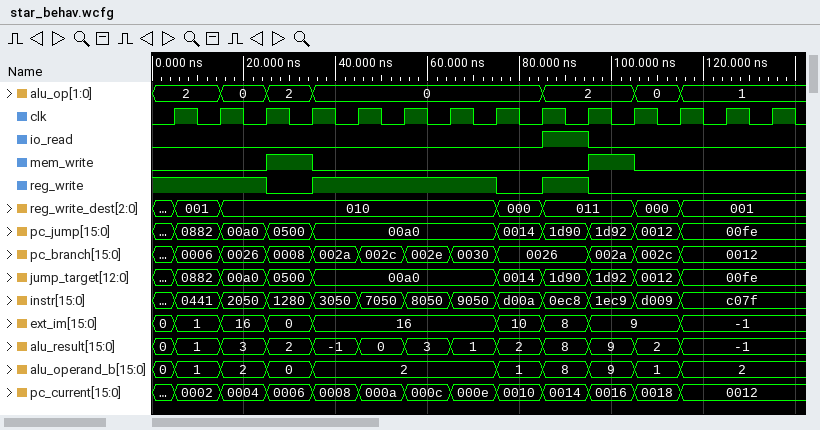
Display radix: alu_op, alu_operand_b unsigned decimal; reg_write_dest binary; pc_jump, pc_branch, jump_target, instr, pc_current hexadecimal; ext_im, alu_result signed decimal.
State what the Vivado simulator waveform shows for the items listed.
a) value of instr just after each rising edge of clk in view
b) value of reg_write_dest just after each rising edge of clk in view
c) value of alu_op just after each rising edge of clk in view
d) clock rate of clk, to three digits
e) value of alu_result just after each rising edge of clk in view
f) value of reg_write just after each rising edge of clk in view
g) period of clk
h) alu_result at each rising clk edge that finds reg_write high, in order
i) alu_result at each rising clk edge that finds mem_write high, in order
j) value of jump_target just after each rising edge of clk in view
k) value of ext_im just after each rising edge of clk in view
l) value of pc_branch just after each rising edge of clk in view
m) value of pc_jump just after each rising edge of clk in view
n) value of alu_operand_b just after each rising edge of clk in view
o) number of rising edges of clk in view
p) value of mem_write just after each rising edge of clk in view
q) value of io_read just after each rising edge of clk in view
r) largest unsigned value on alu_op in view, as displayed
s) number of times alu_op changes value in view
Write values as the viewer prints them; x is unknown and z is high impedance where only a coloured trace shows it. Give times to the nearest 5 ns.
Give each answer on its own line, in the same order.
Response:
0441, 2050, 1280, 3050, 7050, 8050, 9050, d00a, 0ec8, 1ec9, d009, c07f, c07f, c07f
001, 010, 010, 010, 010, 010, 010, 000, 011, 011, 000, 001, 001, 001
2, 0, 2, 0, 0, 0, 0, 0, 2, 2, 0, 1, 1, 1
100 MHz
1, 3, 2, -1, 0, 3, 1, 2, 8, 9, 2, -1, -1, -1
1 1 0 1 1 1 1 0 1 0 0 0 0 0
10 ns
0, 1, 3, -1, 0, 3, 1, 8
2, 9
0882, 00a0, 0500, 00a0, 00a0, 00a0, 00a0, 0014, 1d90, 1d92, 0012, 00fe, 00fe, 00fe
1, 16, 0, 16, 16, 16, 16, 10, 8, 9, 9, -1, -1, -1
0006, 0026, 0008, 002a, 002c, 002e, 0030, 0026, 0026, 002a, 002c, 0012, 0012, 0012
0882, 00a0, 0500, 00a0, 00a0, 00a0, 00a0, 0014, 1d90, 1d92, 0012, 00fe, 00fe, 00fe
1, 2, 0, 2, 2, 2, 2, 1, 8, 9, 1, 2, 2, 2
14
0 0 1 0 0 0 0 0 0 1 0 0 0 0
0 0 0 0 0 0 0 0 1 0 0 0 0 0
2
6
